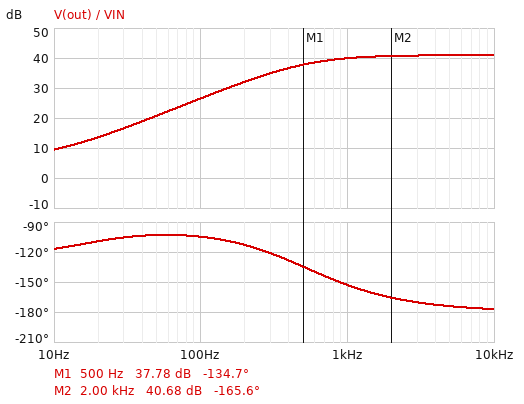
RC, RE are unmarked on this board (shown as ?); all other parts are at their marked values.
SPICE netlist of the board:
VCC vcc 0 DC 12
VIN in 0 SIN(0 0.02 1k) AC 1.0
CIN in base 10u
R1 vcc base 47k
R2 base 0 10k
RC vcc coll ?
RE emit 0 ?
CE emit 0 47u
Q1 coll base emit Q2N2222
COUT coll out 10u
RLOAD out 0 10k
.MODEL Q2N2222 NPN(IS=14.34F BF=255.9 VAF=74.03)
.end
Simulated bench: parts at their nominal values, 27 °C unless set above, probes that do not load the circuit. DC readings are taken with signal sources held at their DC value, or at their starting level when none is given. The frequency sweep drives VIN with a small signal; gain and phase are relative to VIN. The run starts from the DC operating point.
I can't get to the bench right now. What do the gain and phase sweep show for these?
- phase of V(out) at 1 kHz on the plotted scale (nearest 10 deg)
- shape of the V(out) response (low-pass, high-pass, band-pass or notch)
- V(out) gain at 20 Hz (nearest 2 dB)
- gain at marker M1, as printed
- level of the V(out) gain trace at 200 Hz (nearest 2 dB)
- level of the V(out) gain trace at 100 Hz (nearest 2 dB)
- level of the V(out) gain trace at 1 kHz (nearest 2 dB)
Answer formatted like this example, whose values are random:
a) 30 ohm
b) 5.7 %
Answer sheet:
a) -150 deg
b) high-pass
c) 14 dB
d) 37.78 dB
e) 32 dB
f) 26 dB
g) 40 dB
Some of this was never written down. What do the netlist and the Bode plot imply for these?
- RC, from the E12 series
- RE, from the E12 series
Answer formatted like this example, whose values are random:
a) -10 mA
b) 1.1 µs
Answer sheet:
a) 820 Ω
b) 330 Ω
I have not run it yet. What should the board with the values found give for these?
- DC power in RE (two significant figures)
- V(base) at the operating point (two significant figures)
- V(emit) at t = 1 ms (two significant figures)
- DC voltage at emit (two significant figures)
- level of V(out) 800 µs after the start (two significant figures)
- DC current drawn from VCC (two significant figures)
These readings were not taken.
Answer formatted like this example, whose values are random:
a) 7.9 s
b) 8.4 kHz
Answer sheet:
a) 5.2 mW
b) 2.0 V
c) 1.3 V
d) 1.3 V
e) 1.4 V
f) 4.2 mA
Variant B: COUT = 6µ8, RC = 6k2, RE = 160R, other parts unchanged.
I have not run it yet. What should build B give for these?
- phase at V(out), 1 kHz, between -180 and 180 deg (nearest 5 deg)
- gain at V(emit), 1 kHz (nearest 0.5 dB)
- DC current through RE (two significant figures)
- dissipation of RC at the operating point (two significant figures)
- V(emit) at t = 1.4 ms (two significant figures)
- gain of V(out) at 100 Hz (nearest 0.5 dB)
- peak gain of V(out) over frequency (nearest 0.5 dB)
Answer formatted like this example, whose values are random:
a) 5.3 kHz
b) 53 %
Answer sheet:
a) -140 deg
b) -19.0 dB
c) 2.0 mA
d) 22 mW
e) 320 mV
f) -1.0 dB
g) 17.0 dB
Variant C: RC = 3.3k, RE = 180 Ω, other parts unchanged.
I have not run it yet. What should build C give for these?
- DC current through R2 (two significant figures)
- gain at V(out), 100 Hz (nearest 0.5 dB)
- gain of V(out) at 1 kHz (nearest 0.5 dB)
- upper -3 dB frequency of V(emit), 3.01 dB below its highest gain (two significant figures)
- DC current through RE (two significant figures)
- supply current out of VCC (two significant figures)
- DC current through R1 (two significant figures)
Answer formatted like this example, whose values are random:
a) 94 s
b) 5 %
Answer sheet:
a) 130 µA
b) 3.5 dB
c) 21.5 dB
d) 1.3 kHz
e) 3.5 mA
f) 3.6 mA
g) 230 µA
